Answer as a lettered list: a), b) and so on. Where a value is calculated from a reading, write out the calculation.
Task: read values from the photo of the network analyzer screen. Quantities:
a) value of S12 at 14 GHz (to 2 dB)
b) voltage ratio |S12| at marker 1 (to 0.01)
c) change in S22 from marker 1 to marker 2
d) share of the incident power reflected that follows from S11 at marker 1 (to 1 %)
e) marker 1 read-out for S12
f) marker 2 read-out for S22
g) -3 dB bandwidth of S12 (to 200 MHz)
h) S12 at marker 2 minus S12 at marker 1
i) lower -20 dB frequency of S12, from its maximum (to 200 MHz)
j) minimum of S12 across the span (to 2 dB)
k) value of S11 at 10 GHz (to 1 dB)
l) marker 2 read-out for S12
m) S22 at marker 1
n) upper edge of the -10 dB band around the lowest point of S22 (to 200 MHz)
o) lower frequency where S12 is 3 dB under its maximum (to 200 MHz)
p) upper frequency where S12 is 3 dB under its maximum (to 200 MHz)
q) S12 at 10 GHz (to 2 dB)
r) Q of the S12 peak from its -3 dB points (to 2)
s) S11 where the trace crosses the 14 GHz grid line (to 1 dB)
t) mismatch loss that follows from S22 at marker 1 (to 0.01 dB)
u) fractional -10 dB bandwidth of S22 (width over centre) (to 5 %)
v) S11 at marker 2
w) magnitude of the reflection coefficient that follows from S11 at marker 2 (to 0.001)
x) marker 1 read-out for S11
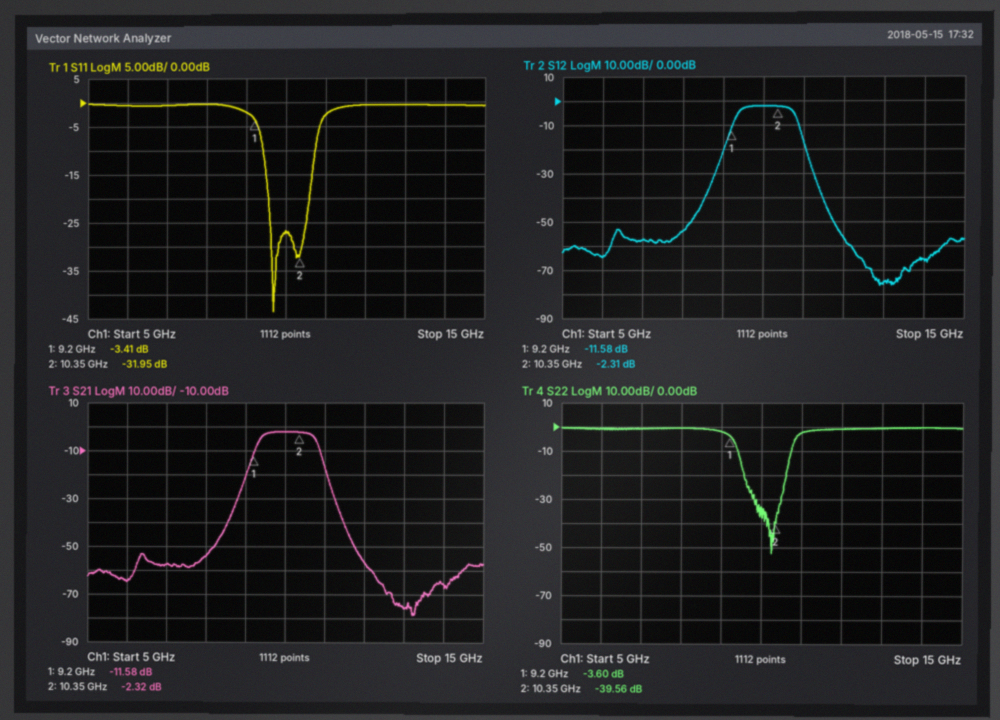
a) -66 dB
b) 10^(-11.58/20) ≈ 0.26
c) -39.56 − (-3.6) = -35.96 dB
d) 10^(-3.41/10) ≈ 46 %
e) -11.58 dB
f) -39.56 dB
g) 10.8 GHz − 9.4 GHz = 1.4 GHz
h) -2.31 − (-11.58) = 9.27 dB
i) 9.0 GHz
j) -76 dB
k) -27 dB
l) -2.31 dB
m) -3.60 dB
n) 10.8 GHz
o) 9.4 GHz
p) 10.8 GHz
q) -2 dB
r) 10.1 GHz / 1.4 GHz ≈ 7.21, so 8 to the nearest 2
s) -1 dB
t) −10 log10(1 − 10^(-3.6/10)) ≈ 2.49 dB
u) 1.4 GHz / 10.1 GHz ≈ 13.9 %, so 15 % to the nearest 5 %
v) -31.95 dB
w) 10^(-31.95/20) ≈ 0.025
x) -3.41 dB
